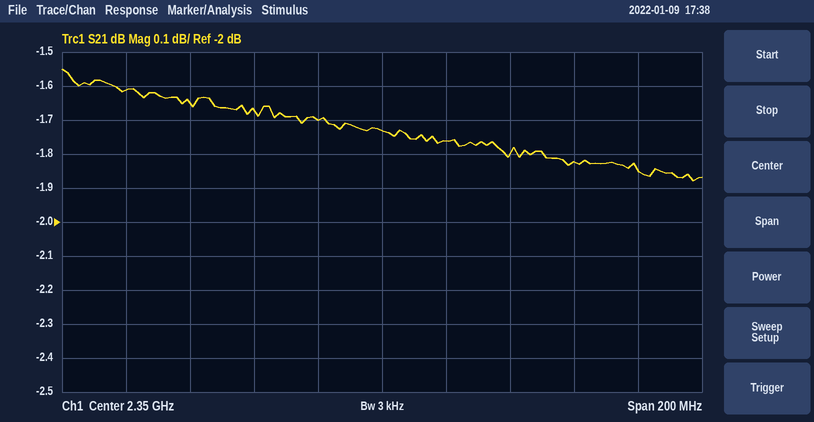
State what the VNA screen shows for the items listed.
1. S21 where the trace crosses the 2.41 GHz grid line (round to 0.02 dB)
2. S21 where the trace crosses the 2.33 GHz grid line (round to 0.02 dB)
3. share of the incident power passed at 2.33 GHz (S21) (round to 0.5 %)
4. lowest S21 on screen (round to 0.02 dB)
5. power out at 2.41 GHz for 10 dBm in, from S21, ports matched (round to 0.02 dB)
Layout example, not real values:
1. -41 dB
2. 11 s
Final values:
1. -1.82 dB
2. -1.70 dB
3. 67.5 %
4. -1.88 dB
5. 8.18 dBm
